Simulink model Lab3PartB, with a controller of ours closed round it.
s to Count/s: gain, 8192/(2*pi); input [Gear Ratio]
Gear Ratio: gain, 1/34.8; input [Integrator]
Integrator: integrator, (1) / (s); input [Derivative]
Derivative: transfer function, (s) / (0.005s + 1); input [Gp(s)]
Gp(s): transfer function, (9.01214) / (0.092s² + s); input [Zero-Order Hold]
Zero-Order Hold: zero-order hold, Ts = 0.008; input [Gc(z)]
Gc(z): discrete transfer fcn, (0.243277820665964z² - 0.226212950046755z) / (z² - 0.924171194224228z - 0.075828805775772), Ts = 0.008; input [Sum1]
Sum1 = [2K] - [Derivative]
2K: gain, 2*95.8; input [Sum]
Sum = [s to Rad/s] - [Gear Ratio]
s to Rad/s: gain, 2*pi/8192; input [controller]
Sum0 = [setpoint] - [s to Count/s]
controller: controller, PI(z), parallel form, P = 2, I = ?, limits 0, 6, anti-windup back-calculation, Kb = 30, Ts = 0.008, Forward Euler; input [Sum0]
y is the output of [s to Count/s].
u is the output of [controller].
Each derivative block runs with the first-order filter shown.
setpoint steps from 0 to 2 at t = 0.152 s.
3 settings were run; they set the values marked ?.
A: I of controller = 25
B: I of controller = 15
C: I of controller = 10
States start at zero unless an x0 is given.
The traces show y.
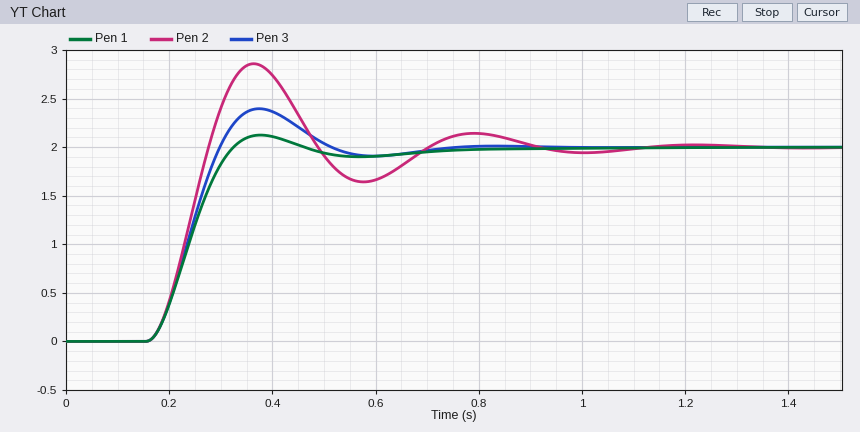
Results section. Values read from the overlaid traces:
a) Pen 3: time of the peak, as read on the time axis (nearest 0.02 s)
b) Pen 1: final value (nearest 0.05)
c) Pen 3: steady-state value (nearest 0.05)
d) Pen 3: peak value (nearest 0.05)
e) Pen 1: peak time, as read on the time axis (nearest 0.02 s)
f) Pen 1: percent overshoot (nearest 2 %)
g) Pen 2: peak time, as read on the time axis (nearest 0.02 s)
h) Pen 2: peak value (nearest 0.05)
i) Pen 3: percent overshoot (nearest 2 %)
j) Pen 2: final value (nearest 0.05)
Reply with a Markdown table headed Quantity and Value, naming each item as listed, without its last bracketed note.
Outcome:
| Quantity | Value |
|---|---|
| Pen 3: time of the peak, as read on the time axis | 0.38 s |
| Pen 1: final value | 2.00 |
| Pen 3: steady-state value | 2.00 |
| Pen 3: peak value | 2.40 |
| Pen 1: peak time, as read on the time axis | 0.38 s |
| Pen 1: percent overshoot | 6 % |
| Pen 2: peak time, as read on the time axis | 0.36 s |
| Pen 2: peak value | 2.85 |
| Pen 3: percent overshoot | 20 % |
| Pen 2: final value | 2.00 |
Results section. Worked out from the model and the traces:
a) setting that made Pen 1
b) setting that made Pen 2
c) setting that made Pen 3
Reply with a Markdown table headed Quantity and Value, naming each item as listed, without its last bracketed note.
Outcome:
| Quantity | Value |
|---|---|
| setting that made Pen 1 | C |
| setting that made Pen 2 | A |
| setting that made Pen 3 | B |
